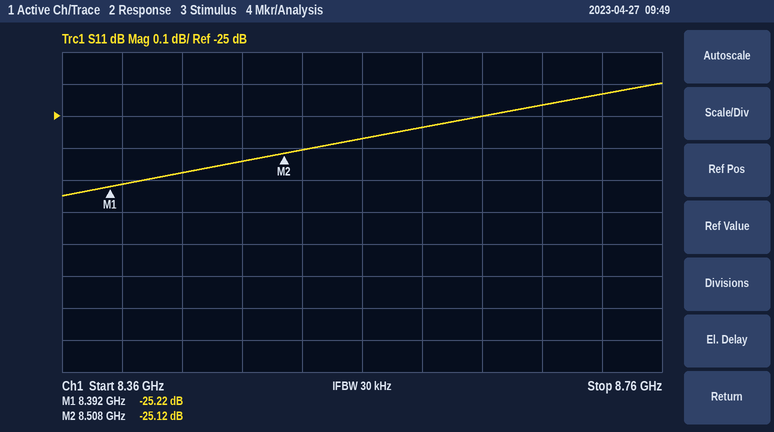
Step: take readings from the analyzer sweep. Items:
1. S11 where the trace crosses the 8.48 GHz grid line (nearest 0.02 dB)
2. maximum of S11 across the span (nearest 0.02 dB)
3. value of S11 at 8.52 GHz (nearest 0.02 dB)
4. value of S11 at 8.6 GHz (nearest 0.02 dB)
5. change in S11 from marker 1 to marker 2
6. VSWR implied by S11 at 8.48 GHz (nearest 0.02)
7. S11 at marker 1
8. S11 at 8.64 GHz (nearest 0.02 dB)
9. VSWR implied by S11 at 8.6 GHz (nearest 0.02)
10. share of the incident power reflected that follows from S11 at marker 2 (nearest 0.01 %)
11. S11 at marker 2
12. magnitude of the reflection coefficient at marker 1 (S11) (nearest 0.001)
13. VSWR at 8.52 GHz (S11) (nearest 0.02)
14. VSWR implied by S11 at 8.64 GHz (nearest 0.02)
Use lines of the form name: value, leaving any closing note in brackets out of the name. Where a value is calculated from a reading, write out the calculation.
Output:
S11 where the trace crosses the 8.48 GHz grid line: -25.14 dB
maximum of S11 across the span: -24.90 dB
value of S11 at 8.52 GHz: -25.10 dB
value of S11 at 8.6 GHz: -25.04 dB
change in S11 from marker 1 to marker 2: -25.12 − (-25.22) = 0.10 dB
VSWR implied by S11 at 8.48 GHz: |Γ| = 10^(-25.14/20) = 0.0553; VSWR = (1 + 0.0553)/(1 − 0.0553) ≈ 1.12
S11 at marker 1: -25.22 dB
S11 at 8.64 GHz: -25.00 dB
VSWR implied by S11 at 8.6 GHz: |Γ| = 10^(-25.04/20) = 0.0560; VSWR = (1 + 0.0560)/(1 − 0.0560) ≈ 1.12
share of the incident power reflected that follows from S11 at marker 2: 10^(-25.12/10) ≈ 0.31 %
S11 at marker 2: -25.12 dB
magnitude of the reflection coefficient at marker 1 (S11): 10^(-25.22/20) ≈ 0.055
VSWR at 8.52 GHz (S11): |Γ| = 10^(-25.1/20) = 0.0556; VSWR = (1 + 0.0556)/(1 − 0.0556) ≈ 1.12
VSWR implied by S11 at 8.64 GHz: |Γ| = 10^(-25/20) = 0.0562; VSWR = (1 + 0.0562)/(1 − 0.0562) ≈ 1.12
